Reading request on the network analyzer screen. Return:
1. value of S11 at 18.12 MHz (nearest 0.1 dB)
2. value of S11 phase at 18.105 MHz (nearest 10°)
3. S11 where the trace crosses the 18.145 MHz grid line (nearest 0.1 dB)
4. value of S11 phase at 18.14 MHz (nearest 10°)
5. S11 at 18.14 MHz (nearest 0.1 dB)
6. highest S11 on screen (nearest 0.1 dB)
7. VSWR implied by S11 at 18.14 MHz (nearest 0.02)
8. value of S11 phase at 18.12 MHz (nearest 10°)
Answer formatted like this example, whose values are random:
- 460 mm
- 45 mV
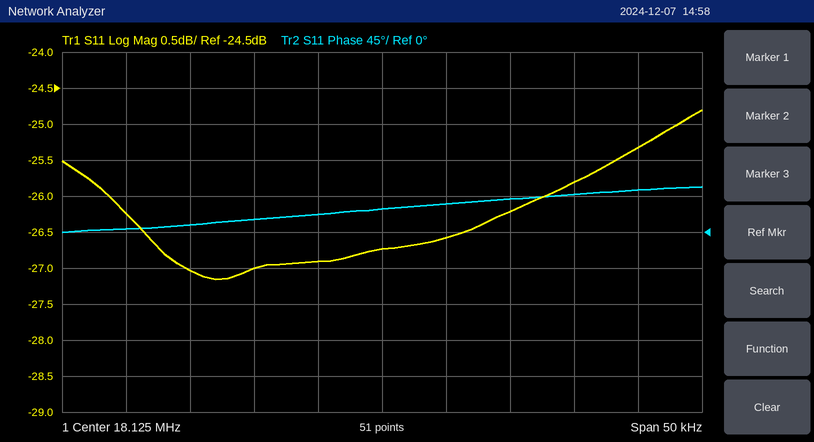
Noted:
- -26.9 dB
- 0°
- -25.3 dB
- 50°
- -25.8 dB
- -24.8 dB
- 1.10
- 20°
